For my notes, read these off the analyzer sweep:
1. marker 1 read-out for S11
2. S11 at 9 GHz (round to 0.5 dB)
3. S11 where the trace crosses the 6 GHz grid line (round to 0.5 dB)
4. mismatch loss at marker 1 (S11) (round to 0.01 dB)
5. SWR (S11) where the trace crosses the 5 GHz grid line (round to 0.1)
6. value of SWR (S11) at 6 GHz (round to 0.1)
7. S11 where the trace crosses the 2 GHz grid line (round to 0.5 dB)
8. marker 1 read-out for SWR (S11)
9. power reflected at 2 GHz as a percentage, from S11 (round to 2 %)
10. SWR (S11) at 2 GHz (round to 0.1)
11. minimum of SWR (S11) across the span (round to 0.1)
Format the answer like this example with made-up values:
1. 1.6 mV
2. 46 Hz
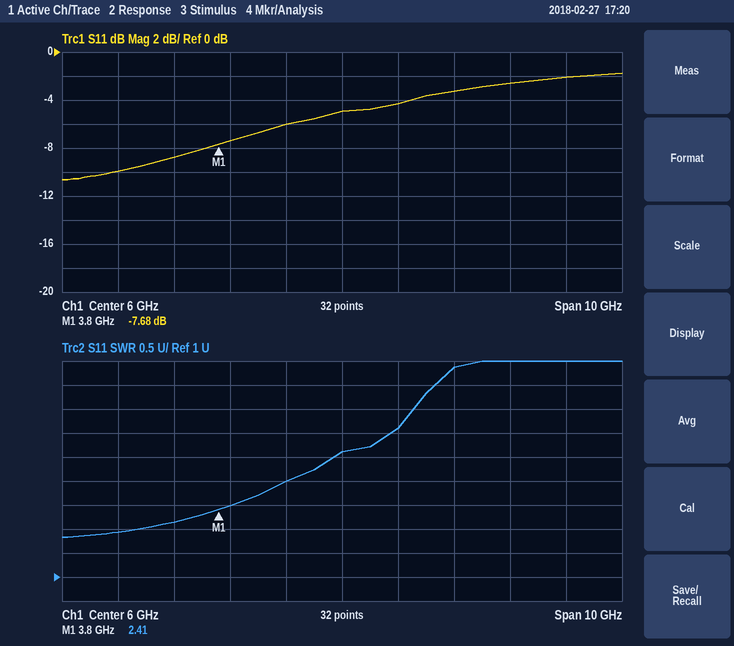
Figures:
1. -7.68 dB
2. -2.5 dB
3. -5.0 dB
4. 0.81 dB
5. 3.0
6. 3.6
7. -10.0 dB
8. 2.41
9. 10 %
10. 1.9
11. 1.8
